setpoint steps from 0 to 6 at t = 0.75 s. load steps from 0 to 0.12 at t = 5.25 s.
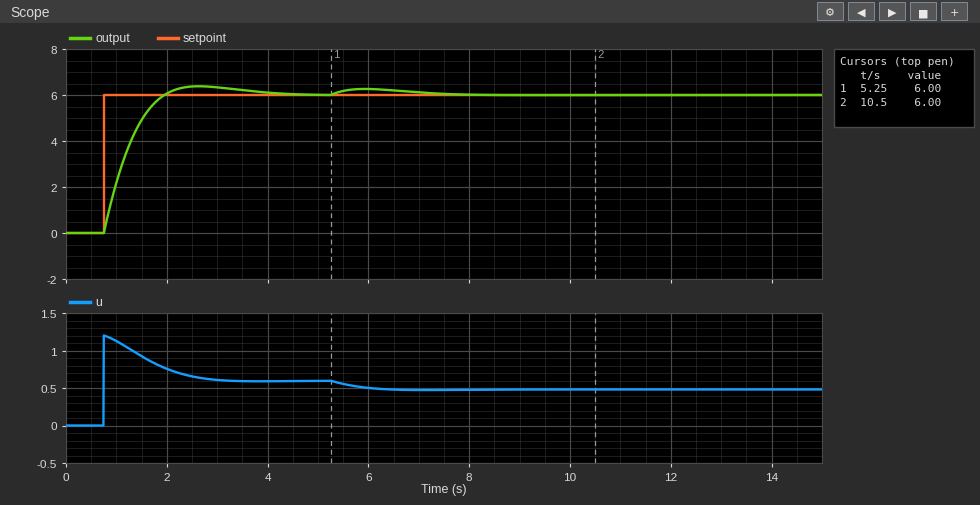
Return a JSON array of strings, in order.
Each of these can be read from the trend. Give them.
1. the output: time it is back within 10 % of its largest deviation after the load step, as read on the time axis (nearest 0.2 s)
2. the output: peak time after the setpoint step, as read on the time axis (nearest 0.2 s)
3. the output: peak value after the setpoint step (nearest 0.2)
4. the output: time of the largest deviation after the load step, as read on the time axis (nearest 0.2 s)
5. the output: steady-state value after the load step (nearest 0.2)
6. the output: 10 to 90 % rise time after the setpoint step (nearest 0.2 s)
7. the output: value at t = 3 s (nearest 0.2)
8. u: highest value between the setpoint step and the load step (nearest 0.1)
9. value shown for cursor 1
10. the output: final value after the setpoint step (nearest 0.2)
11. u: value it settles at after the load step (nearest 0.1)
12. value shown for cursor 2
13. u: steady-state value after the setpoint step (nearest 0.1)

["7.8 s", "2.6 s", "6.4", "6.0 s", "6.0", "0.8 s", "6.4", "1.2", "6.00", "6.0", "0.5", "6.00", "0.6"]
